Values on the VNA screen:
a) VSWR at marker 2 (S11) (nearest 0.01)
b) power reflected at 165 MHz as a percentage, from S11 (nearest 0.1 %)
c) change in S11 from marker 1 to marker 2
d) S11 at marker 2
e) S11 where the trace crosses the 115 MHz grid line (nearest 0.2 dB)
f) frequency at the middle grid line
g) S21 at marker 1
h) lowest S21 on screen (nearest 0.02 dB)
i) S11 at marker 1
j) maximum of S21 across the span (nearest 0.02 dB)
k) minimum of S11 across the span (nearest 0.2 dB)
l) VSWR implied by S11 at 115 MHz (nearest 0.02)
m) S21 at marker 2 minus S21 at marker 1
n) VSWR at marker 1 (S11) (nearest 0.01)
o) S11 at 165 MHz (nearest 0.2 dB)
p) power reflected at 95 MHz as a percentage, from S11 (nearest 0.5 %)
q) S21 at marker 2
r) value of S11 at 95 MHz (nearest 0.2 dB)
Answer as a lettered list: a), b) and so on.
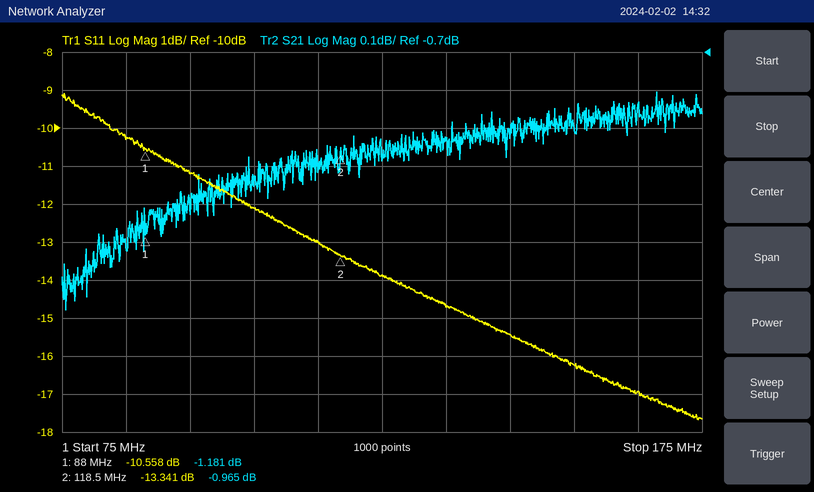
a) 1.55
b) 2.0 %
c) -2.783 dB
d) -13.341 dB
e) -13.0 dB
f) 125 MHz
g) -1.181 dB
h) -1.38 dB
i) -10.558 dB
j) -0.80 dB
k) -17.6 dB
l) 1.58
m) 0.216 dB
n) 1.84
o) -17.0 dB
p) 7.5 %
q) -0.965 dB
r) -11.2 dB
